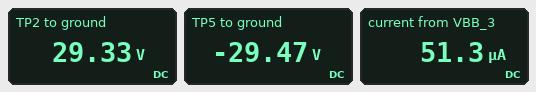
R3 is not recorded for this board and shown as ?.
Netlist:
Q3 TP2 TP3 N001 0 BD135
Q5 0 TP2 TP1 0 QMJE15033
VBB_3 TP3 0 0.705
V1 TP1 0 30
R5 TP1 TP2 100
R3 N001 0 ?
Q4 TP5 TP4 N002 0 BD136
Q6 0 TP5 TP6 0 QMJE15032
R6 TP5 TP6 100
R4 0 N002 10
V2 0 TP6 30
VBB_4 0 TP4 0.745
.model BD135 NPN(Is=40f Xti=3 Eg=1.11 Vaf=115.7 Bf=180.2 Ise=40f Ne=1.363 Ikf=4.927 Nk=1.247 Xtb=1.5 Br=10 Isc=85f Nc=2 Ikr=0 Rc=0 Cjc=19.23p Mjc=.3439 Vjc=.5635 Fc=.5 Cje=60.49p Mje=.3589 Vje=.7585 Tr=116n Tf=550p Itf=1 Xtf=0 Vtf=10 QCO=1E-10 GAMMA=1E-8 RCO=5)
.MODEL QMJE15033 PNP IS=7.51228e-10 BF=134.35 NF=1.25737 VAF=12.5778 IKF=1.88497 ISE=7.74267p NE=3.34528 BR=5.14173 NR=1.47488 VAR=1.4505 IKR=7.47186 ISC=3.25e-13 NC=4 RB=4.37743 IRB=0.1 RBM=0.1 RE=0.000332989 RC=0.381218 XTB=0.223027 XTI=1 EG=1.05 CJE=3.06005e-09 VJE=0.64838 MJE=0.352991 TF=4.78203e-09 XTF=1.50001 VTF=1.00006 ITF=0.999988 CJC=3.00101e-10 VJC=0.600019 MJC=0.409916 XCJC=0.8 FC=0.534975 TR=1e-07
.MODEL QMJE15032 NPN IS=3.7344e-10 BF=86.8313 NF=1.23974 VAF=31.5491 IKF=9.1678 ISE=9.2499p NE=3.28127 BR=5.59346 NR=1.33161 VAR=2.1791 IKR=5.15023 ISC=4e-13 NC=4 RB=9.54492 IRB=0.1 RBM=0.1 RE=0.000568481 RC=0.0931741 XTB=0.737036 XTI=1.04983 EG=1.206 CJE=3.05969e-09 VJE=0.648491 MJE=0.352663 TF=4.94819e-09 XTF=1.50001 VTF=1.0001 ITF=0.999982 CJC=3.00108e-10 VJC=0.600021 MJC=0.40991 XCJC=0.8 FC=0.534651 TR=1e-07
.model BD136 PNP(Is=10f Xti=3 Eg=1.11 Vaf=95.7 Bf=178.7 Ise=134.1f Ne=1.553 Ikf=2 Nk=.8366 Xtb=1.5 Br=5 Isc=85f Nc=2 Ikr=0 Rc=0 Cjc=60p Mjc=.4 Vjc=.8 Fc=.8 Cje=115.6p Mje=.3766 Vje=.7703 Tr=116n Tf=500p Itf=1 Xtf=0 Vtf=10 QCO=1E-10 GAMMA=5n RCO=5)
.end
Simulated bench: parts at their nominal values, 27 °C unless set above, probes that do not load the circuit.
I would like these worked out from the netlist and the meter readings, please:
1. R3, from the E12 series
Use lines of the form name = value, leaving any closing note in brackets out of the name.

R3, from the E12 series = 3.3 Ω
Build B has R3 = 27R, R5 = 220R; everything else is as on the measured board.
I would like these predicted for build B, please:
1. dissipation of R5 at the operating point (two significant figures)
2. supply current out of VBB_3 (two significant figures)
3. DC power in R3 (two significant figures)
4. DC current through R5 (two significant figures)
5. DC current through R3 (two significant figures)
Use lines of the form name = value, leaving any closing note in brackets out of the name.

dissipation of R5 at the operating point = 1.3 mW
supply current out of VBB_3 = 14 µA
DC power in R3 = 170 µW
DC current through R5 = 2.4 mA
DC current through R3 = 2.5 mA
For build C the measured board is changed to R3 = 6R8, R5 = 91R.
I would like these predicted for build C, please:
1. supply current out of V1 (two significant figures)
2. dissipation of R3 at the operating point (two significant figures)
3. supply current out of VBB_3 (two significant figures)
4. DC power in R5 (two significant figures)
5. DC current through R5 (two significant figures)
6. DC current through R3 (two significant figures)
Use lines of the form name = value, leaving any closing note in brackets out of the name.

supply current out of V1 = 77 mA
dissipation of R3 at the operating point = 280 µW
supply current out of VBB_3 = 34 µA
DC power in R5 = 3.5 mW
DC current through R5 = 6.2 mA
DC current through R3 = 6.4 mA
